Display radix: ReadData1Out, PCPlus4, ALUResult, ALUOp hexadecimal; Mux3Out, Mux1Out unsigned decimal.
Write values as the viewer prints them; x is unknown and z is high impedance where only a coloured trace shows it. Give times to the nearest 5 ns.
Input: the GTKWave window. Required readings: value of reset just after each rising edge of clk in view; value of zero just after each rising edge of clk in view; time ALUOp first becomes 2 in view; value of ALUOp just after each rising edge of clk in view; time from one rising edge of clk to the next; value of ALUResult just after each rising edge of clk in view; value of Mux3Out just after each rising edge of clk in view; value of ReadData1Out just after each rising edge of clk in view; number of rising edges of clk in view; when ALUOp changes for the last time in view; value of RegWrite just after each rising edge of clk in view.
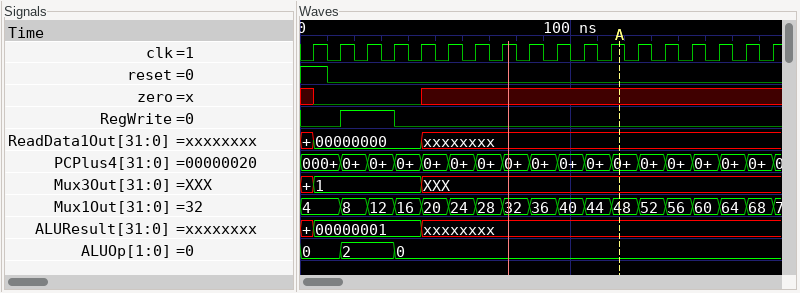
1 0 0 0 0 0 0 0 0 0 0 0 0 0 0 0 0 0
0 0 0 0 x x x x x x x x x x x x x x
15 ns
0, 2, 2, 0, 0, 0, 0, 0, 0, 0, 0, 0, 0, 0, 0, 0, 0, 0
10 ns
00000001, 00000001, 00000001, 00000001, xxxxxxxx, xxxxxxxx, xxxxxxxx, xxxxxxxx, xxxxxxxx, xxxxxxxx, xxxxxxxx, xxxxxxxx, xxxxxxxx, xxxxxxxx, xxxxxxxx, xxxxxxxx, xxxxxxxx, xxxxxxxx
1, 1, 1, 1, XXX, XXX, XXX, XXX, XXX, XXX, XXX, XXX, XXX, XXX, XXX, XXX, XXX, XXX
00000000, 00000000, 00000000, 00000000, xxxxxxxx, xxxxxxxx, xxxxxxxx, xxxxxxxx, xxxxxxxx, xxxxxxxx, xxxxxxxx, xxxxxxxx, xxxxxxxx, xxxxxxxx, xxxxxxxx, xxxxxxxx, xxxxxxxx, xxxxxxxx
18
35 ns
0 1 1 0 0 0 0 0 0 0 0 0 0 0 0 0 0 0
